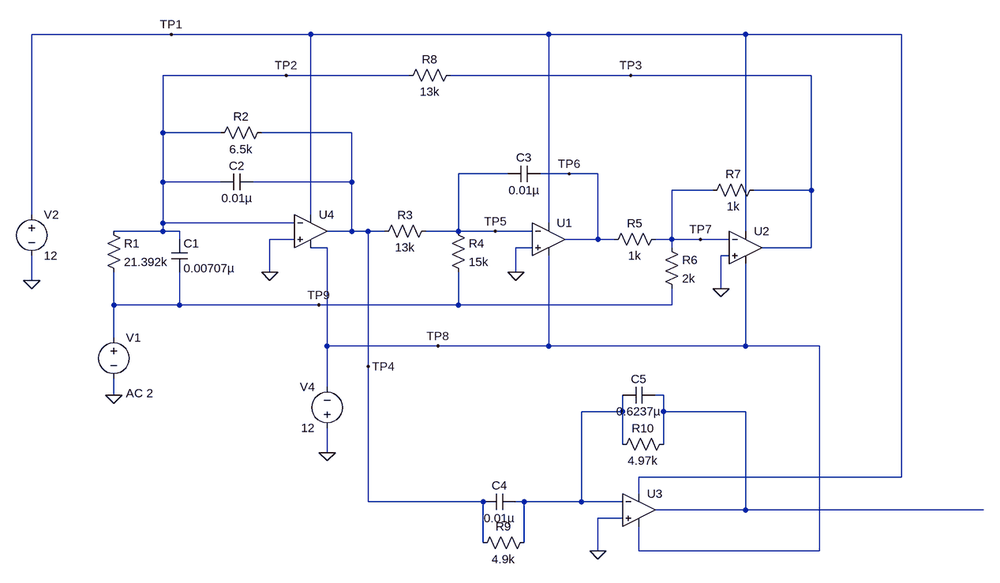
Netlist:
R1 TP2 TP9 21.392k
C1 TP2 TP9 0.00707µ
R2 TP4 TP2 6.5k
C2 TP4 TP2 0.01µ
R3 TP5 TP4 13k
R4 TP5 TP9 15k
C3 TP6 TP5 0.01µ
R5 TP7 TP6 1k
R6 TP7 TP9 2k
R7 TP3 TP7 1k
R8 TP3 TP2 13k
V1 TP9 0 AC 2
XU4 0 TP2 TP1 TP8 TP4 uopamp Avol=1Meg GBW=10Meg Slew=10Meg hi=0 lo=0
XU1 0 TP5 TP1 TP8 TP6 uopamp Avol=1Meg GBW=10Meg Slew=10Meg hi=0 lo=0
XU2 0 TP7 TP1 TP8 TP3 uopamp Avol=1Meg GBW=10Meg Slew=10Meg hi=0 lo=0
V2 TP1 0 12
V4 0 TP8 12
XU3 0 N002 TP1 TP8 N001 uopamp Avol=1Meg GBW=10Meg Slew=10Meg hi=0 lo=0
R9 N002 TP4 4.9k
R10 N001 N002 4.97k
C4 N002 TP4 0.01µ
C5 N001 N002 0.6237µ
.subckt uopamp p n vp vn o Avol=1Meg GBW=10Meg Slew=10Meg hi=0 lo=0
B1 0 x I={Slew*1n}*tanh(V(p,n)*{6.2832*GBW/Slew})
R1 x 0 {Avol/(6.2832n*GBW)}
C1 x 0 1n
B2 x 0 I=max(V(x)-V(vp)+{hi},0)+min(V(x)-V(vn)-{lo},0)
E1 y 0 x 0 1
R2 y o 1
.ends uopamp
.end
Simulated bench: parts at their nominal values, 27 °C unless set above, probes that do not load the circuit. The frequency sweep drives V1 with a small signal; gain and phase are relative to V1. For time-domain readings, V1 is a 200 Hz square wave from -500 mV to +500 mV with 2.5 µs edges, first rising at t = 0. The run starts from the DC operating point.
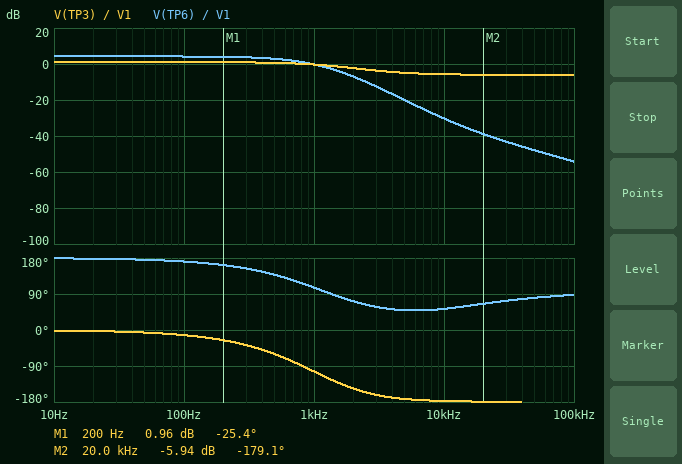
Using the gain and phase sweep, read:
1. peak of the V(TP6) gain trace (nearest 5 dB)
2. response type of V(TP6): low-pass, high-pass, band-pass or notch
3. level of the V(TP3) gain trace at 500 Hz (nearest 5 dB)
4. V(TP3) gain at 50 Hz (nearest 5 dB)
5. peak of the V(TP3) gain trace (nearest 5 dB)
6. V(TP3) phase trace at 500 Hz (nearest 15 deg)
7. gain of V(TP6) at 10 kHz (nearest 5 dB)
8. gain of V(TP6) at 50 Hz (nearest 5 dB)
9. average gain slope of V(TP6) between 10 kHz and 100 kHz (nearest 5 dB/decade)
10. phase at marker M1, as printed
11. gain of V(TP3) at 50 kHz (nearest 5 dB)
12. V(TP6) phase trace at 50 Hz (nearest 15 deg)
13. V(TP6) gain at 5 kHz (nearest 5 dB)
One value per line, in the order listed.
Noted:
5 dB
low-pass
0 dB
0 dB
0 dB
-60 deg
-30 dB
5 dB
-25 dB/decade
-25.4 deg
-5 dB
180 deg
-20 dB
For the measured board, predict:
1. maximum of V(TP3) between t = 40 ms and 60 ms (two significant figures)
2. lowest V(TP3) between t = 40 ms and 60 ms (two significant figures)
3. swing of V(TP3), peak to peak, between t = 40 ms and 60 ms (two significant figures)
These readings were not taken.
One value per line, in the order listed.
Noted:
1.1 V
-1.1 V
2.1 V
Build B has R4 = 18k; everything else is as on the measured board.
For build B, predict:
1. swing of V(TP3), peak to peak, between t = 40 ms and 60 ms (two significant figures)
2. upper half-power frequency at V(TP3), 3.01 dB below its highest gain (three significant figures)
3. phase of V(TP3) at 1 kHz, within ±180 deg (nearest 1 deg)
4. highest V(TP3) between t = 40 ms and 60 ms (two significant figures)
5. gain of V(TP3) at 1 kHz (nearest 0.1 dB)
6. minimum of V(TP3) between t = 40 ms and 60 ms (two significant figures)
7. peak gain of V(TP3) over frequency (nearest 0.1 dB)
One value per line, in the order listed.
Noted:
1.8 V
3.63 kHz
-113 deg
920 mV
-1.4 dB
-920 mV
-1.3 dB
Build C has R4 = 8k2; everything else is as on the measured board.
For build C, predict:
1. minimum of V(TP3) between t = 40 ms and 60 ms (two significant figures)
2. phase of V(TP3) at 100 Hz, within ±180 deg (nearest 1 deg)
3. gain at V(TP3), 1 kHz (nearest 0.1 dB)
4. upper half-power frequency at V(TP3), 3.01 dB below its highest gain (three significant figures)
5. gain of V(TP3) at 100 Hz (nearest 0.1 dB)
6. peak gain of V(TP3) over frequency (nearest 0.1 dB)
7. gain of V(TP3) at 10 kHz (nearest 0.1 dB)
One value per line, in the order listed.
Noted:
-1.8 V
-10 deg
4.8 dB
927 Hz
8.1 dB
8.2 dB
-5.5 dB
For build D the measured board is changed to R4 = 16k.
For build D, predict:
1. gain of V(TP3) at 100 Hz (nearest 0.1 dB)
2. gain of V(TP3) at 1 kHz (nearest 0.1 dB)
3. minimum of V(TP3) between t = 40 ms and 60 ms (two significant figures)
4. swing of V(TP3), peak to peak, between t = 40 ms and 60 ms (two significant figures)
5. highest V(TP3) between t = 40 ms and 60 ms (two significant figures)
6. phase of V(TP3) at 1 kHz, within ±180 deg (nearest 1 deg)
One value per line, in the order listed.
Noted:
0.1 dB
-0.7 dB
-1.0 V
2.0 V
1.0 V
-107 deg
